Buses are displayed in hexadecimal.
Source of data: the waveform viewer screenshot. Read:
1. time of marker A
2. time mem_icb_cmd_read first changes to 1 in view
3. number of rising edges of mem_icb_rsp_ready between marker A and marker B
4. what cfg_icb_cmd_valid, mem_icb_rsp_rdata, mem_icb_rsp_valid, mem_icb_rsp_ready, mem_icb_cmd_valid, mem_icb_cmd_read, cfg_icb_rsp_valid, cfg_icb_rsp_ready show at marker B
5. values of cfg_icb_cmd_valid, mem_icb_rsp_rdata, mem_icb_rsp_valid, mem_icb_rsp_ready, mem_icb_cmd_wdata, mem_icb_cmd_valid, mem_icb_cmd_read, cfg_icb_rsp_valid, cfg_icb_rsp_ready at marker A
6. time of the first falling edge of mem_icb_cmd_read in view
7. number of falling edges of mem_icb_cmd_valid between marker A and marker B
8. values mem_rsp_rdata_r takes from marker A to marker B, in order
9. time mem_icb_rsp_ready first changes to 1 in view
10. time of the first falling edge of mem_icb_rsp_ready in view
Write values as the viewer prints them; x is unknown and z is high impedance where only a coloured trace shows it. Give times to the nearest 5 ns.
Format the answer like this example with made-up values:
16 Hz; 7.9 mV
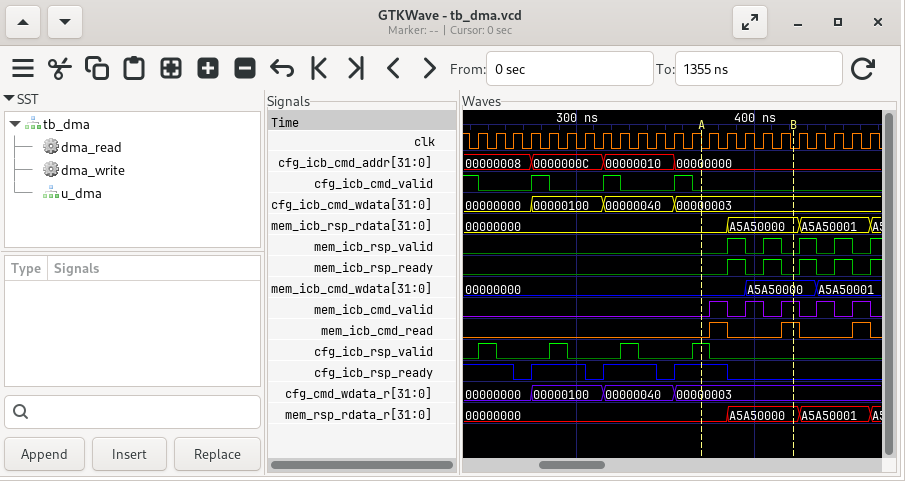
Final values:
370 ns; 375 ns; 2; cfg_icb_cmd_valid=0, mem_icb_rsp_rdata=A5A50000, mem_icb_rsp_valid=0, mem_icb_rsp_ready=0, mem_icb_cmd_valid=1, mem_icb_cmd_read=1, cfg_icb_rsp_valid=0, cfg_icb_rsp_ready=0; cfg_icb_cmd_valid=0, mem_icb_rsp_rdata=00000000, mem_icb_rsp_valid=0, mem_icb_rsp_ready=0, mem_icb_cmd_wdata=00000000, mem_icb_cmd_valid=0, mem_icb_cmd_read=0, cfg_icb_rsp_valid=1, cfg_icb_rsp_ready=1; 385 ns; 2; 00000000, A5A50000; 385 ns; 395 ns
